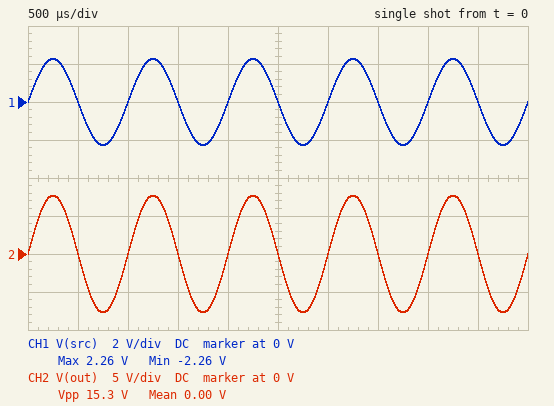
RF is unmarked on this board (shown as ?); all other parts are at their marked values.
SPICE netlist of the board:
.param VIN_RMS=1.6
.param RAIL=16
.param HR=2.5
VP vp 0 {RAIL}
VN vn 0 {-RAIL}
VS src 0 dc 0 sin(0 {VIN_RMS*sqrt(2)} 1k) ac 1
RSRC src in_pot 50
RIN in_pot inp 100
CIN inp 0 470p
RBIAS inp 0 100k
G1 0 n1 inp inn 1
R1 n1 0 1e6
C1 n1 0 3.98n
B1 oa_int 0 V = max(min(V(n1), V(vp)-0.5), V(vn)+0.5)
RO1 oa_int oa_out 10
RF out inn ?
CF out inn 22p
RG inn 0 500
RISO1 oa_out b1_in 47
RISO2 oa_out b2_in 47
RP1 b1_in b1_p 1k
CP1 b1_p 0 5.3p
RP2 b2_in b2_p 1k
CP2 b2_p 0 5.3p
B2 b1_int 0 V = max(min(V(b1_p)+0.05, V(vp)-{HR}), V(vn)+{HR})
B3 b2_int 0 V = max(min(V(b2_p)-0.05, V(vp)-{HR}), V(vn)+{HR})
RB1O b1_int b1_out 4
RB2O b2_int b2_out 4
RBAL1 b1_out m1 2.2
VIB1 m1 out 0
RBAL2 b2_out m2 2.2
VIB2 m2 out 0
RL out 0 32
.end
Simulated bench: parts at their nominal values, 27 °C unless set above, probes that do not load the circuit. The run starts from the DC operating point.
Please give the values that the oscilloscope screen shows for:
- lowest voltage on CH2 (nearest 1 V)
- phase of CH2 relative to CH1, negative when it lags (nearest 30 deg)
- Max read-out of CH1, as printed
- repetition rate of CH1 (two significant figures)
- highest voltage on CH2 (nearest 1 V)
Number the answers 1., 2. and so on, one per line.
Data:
1. -8 V
2. 0 deg
3. 2.26 V
4. 1.0 kHz
5. 8 V
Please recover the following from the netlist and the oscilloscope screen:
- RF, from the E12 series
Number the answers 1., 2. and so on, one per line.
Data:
1. 1.2 kΩ
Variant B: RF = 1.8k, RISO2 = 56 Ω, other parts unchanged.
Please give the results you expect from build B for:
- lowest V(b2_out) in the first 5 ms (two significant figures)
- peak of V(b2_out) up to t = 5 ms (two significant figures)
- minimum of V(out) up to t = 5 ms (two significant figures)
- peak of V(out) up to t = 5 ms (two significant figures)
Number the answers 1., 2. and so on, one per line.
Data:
1. -11 V
2. 11 V
3. -10 V
4. 10 V
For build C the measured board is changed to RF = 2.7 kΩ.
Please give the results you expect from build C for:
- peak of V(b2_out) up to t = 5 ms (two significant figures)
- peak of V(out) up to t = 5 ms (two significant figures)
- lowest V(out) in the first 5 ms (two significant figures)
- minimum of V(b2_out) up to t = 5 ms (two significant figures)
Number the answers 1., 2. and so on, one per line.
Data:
1. 13 V
2. 12 V
3. -12 V
4. -13 V
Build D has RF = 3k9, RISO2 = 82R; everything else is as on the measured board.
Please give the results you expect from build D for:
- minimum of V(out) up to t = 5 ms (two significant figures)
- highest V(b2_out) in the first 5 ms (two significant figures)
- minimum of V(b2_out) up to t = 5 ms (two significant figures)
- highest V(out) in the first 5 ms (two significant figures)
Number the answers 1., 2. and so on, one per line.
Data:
1. -12 V
2. 13 V
3. -13 V
4. 12 V
